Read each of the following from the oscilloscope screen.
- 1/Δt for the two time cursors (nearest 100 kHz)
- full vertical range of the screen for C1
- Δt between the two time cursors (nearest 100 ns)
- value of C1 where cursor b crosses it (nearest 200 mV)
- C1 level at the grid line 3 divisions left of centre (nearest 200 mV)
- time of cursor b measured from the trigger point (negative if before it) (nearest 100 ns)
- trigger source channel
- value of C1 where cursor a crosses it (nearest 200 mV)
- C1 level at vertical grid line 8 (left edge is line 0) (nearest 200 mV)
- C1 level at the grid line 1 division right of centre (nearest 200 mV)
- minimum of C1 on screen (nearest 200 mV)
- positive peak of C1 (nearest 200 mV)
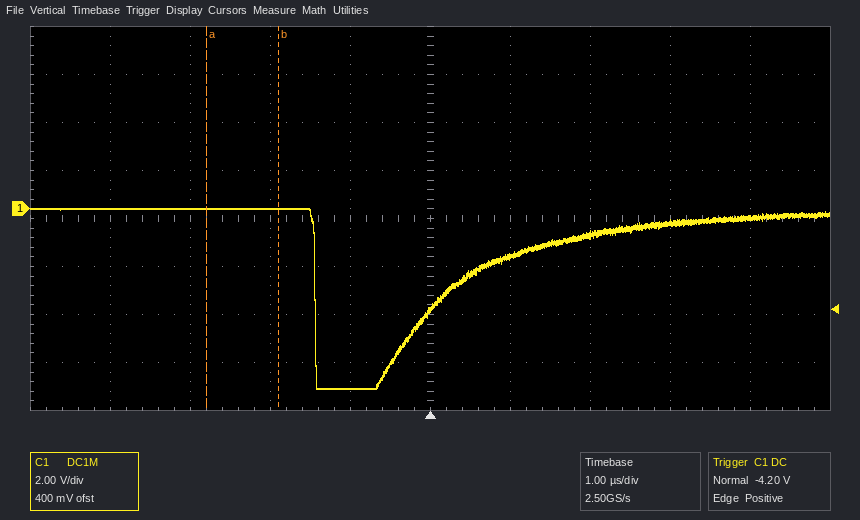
1.1 MHz
16 V
900 ns
0.0 V
0.0 V
-1.9 µs
C1
0.0 V
-600 mV
-2.0 V
-7.4 V
0.0 V
